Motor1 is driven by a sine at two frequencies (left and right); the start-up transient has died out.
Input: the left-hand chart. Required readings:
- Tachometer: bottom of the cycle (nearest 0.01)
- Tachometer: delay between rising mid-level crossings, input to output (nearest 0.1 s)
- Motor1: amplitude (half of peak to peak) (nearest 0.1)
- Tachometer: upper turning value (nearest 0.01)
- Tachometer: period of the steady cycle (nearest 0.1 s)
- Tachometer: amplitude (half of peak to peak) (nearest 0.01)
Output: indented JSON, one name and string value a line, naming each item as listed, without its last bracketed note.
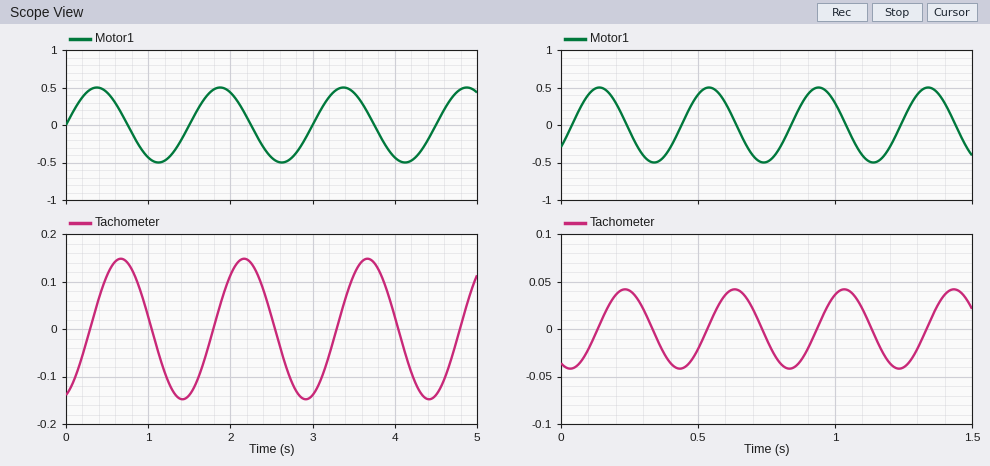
{
  "Tachometer: bottom of the cycle": "-0.15",
  "Tachometer: delay between rising mid-level crossings, input to output": "0.3 s",
  "Motor1: amplitude (half of peak to peak)": "0.5",
  "Tachometer: upper turning value": "0.15",
  "Tachometer: period of the steady cycle": "1.5 s",
  "Tachometer: amplitude (half of peak to peak)": "0.15"
}
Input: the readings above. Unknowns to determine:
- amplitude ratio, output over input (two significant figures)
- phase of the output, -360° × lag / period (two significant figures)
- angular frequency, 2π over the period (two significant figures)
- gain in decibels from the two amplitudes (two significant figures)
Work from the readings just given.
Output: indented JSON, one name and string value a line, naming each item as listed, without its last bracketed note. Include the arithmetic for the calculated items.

{
  "amplitude ratio, output over input": "0.15 / 0.5 = 0.30",
  "phase of the output, -360° × lag / period": "-360 × 0.3 / 1.5 = -72°",
  "angular frequency, 2π over the period": "2π / 1.5 = 4.2 rad/s",
  "gain in decibels from the two amplitudes": "20 log10(0.15 / 0.5) = -10 dB"
}
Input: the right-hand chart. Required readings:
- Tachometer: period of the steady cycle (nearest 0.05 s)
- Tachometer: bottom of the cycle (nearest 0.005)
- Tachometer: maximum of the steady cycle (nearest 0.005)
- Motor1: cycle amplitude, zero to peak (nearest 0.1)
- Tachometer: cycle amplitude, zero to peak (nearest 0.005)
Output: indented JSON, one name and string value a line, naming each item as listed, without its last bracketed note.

{
  "Tachometer: period of the steady cycle": "0.40 s",
  "Tachometer: bottom of the cycle": "-0.040",
  "Tachometer: maximum of the steady cycle": "0.040",
  "Motor1: cycle amplitude, zero to peak": "0.5",
  "Tachometer: cycle amplitude, zero to peak": "0.040"
}
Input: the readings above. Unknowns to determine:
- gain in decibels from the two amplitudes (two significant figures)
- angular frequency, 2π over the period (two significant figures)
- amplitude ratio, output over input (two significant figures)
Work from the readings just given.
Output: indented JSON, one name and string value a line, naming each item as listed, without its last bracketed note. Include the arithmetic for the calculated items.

{
  "gain in decibels from the two amplitudes": "20 log10(0.04 / 0.5) = -22 dB",
  "angular frequency, 2π over the period": "2π / 0.4 = 16 rad/s",
  "amplitude ratio, output over input": "0.04 / 0.5 = 0.080"
}
